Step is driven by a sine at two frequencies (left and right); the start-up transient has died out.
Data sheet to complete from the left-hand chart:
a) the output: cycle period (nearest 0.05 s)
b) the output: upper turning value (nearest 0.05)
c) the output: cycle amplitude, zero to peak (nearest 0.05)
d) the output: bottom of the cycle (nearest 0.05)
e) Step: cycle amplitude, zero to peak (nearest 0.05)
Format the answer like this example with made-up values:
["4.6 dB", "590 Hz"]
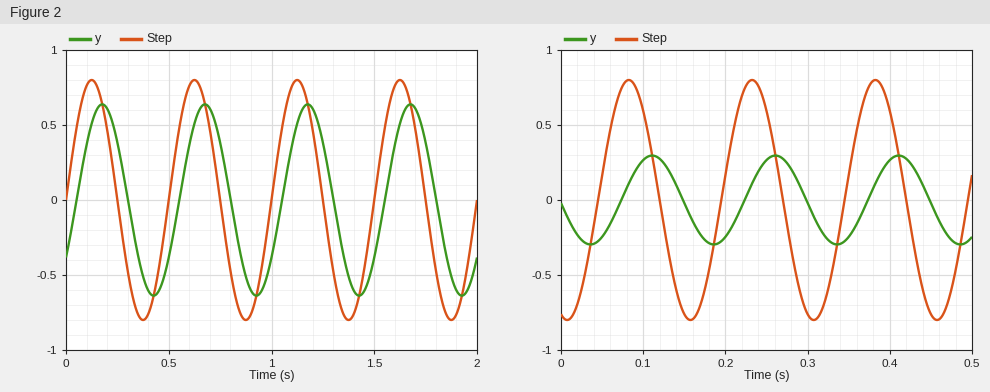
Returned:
["0.50 s", "0.65", "0.65", "-0.65", "0.80"]
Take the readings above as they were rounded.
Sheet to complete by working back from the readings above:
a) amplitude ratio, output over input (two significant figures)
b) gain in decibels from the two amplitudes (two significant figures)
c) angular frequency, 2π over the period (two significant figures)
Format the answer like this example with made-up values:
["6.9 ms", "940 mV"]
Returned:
["0.81", "-1.8 dB", "13 rad/s"]
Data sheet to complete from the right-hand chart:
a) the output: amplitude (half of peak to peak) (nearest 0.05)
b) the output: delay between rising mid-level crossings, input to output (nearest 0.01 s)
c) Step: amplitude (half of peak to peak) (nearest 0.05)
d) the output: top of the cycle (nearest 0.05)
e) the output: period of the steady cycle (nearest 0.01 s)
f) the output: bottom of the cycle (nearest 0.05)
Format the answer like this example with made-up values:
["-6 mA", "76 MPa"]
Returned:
["0.30", "0.03 s", "0.80", "0.30", "0.15 s", "-0.30"]
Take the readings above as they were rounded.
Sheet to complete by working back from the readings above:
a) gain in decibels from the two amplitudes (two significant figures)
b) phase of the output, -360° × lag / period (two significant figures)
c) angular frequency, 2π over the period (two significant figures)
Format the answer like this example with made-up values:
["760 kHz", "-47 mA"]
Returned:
["-8.5 dB", "-72°", "42 rad/s"]
